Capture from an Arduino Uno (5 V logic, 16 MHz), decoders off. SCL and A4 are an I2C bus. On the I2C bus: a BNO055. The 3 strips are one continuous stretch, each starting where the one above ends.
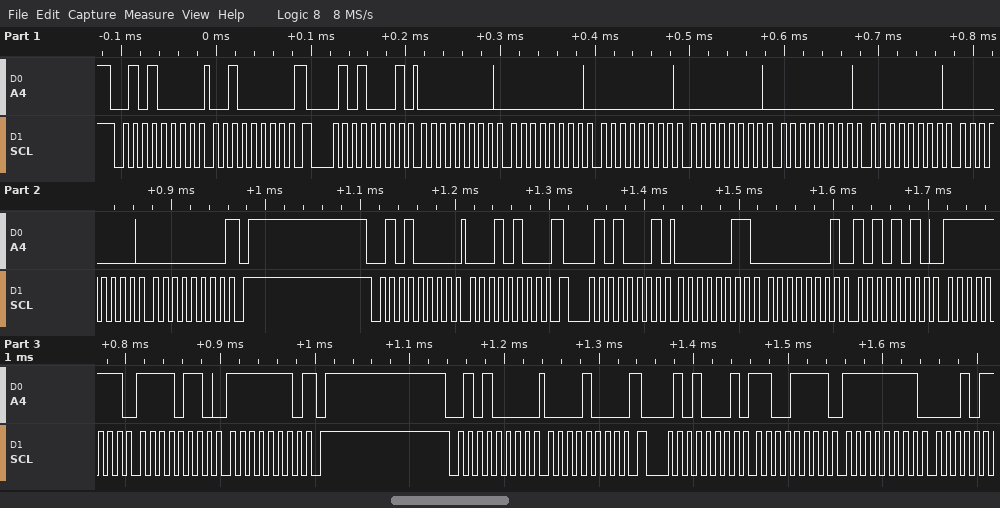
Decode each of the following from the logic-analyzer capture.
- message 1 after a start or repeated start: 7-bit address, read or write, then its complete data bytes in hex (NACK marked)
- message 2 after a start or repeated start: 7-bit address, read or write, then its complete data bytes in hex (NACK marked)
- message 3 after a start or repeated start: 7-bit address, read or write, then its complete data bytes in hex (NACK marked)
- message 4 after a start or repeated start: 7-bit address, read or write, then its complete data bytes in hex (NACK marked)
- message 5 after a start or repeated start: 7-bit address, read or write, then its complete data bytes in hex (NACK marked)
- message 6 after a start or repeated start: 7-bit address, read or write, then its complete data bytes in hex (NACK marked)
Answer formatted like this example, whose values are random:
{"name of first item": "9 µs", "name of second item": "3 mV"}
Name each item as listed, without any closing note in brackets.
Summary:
{"message 1 after a start or repeated start: 7-bit address, read or write, then its complete data bytes in hex": "0x28 write: 20", "message 2 after a start or repeated start: 7-bit address, read or write, then its complete data bytes in hex": "0x28 read: 00 00 00 00 00 00 00 00 NACK", "message 3 after a start or repeated start: 7-bit address, read or write, then its complete data bytes in hex": "0x28 write: 14", "message 4 after a start or repeated start: 7-bit address, read or write, then its complete data bytes in hex": "0x28 read: 03 01 AA FF F6 FE NACK", "message 5 after a start or repeated start: 7-bit address, read or write, then its complete data bytes in hex": "0x28 write: 08", "message 6 after a start or repeated start: 7-bit address, read or write, then its complete data bytes in hex": "0x28 read: CF FF"}
